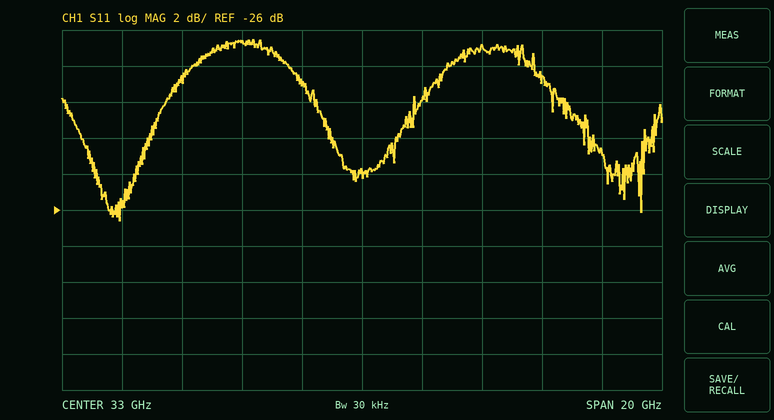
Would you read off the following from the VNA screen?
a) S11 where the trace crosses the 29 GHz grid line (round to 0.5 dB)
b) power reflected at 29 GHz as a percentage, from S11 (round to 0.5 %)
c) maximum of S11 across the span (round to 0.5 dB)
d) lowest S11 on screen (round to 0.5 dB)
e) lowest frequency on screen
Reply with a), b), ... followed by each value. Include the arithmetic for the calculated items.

a) -16.5 dB
b) 10^(-16.5/10) ≈ 2.24 %, so 2.0 % to the nearest 0.5 %
c) -16.5 dB
d) -26.5 dB
e) 23 GHz
